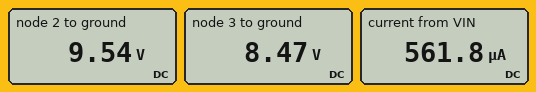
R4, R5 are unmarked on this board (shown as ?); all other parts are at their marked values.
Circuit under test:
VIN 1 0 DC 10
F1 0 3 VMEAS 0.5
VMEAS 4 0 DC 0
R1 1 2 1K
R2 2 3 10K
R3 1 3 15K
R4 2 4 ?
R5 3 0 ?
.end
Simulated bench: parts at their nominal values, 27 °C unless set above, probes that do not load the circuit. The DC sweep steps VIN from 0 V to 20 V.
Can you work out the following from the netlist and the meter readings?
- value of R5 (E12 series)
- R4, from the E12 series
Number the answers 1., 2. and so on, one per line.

1. 22 kΩ
2. 27 kΩ
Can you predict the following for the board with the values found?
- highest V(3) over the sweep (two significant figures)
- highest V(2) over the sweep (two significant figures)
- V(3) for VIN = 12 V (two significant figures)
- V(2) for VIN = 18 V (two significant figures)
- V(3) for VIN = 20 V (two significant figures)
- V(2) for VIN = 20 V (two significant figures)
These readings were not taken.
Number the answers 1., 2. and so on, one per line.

1. 17 V
2. 19 V
3. 10 V
4. 17 V
5. 17 V
6. 19 V
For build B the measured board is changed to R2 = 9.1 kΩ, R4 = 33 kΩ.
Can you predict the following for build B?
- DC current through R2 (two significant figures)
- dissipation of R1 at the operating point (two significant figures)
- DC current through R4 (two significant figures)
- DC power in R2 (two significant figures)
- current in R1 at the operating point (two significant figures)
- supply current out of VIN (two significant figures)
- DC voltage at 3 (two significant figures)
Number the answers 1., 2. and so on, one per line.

1. 130 µA
2. 180 µW
3. 290 µA
4. 150 µW
5. 420 µA
6. 530 µA
7. 8.4 V
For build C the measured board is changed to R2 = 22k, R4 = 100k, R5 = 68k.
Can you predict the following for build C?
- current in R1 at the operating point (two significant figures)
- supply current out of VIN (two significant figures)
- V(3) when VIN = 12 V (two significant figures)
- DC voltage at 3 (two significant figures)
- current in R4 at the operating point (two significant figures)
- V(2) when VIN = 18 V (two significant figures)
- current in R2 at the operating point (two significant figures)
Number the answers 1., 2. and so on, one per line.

1. 130 µA
2. 180 µA
3. 11 V
4. 9.2 V
5. 99 µA
6. 18 V
7. 31 µA
